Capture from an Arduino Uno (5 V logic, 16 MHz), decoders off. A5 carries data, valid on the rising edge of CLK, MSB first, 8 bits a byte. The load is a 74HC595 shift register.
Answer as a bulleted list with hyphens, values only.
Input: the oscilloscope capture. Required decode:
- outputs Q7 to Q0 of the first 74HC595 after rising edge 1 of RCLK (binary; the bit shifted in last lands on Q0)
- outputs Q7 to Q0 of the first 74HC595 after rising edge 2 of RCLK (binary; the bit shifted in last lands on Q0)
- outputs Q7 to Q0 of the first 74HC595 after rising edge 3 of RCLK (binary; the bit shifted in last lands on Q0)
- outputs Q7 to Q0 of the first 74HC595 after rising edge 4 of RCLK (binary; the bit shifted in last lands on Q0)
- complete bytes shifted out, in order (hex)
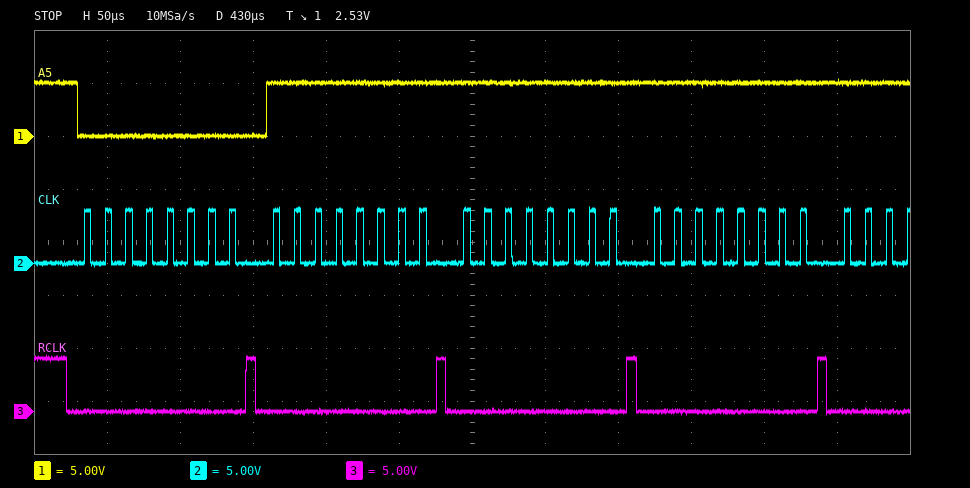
- 00000000
- 11111111
- 11111111
- 11111111
- 0x00 0xFF 0xFF 0xFF
